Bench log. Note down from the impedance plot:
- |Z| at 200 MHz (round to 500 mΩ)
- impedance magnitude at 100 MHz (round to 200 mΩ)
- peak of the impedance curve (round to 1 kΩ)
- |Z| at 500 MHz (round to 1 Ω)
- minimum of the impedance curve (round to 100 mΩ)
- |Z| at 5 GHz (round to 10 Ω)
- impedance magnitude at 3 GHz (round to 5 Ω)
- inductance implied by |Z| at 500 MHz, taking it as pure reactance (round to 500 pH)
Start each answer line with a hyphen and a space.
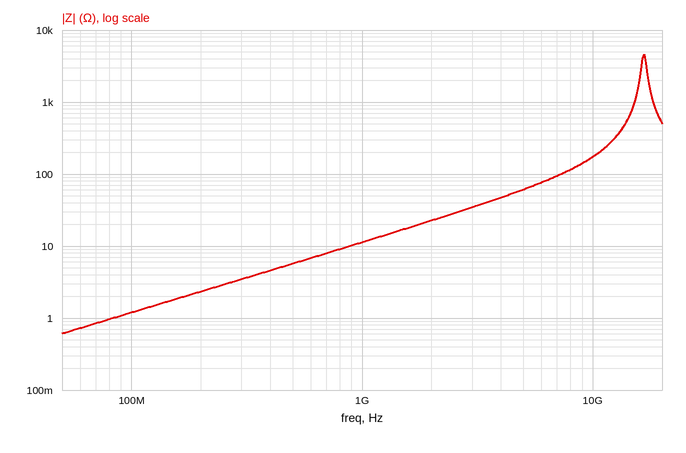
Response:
- 2.5 Ω
- 1.2 Ω
- 5 kΩ
- 6 Ω
- 600 mΩ
- 60 Ω
- 35 Ω
- 2.0 nH
